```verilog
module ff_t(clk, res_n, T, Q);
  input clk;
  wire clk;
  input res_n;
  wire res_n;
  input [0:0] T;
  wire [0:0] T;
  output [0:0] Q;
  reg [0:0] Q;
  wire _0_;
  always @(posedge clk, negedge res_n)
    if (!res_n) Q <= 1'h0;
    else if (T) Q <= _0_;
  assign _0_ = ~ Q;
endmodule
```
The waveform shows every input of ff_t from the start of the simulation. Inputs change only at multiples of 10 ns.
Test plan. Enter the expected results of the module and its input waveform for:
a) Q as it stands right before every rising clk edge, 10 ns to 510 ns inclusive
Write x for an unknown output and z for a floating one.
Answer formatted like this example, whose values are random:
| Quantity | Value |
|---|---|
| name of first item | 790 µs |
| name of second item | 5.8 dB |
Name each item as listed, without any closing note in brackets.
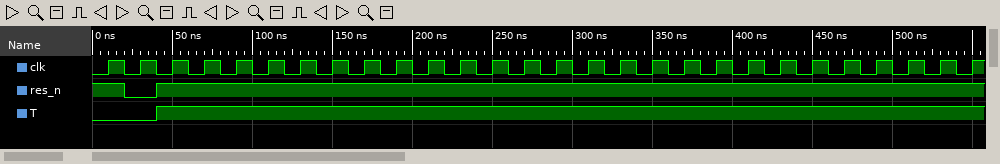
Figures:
| Quantity | Value |
|---|---|
| Q as it stands right before every rising clk edge, 10 ns to 510 ns inclusive | x 0 0 1 0 1 0 1 0 1 0 1 0 1 0 1 0 1 0 1 0 1 0 1 0 1 |
